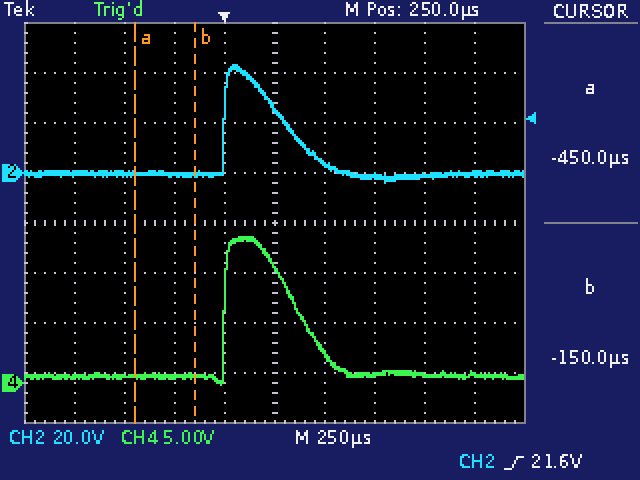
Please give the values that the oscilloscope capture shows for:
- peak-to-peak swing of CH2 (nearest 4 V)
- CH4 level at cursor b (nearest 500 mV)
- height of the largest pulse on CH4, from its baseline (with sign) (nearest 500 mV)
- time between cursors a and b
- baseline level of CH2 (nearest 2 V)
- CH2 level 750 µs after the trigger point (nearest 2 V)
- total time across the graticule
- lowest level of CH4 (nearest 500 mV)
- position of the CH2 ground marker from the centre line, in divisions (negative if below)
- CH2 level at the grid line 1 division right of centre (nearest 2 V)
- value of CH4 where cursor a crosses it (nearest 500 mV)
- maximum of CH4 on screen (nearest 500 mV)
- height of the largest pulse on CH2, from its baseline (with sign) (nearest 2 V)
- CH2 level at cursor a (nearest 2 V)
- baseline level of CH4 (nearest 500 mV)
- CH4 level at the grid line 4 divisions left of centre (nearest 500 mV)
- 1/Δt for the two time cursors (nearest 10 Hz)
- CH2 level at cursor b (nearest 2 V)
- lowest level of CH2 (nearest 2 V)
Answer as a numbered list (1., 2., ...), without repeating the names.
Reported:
1. 48 V
2. 500 mV
3. +14.0 V
4. 300 µs
5. 0 V
6. -2 V
7. 2.5 ms
8. 0.0 V
9. +1.0 div
10. 4 V
11. 500 mV
12. 14.5 V
13. +44 V
14. 0 V
15. 500 mV
16. 500 mV
17. 3.33 kHz
18. 0 V
19. -4 V
